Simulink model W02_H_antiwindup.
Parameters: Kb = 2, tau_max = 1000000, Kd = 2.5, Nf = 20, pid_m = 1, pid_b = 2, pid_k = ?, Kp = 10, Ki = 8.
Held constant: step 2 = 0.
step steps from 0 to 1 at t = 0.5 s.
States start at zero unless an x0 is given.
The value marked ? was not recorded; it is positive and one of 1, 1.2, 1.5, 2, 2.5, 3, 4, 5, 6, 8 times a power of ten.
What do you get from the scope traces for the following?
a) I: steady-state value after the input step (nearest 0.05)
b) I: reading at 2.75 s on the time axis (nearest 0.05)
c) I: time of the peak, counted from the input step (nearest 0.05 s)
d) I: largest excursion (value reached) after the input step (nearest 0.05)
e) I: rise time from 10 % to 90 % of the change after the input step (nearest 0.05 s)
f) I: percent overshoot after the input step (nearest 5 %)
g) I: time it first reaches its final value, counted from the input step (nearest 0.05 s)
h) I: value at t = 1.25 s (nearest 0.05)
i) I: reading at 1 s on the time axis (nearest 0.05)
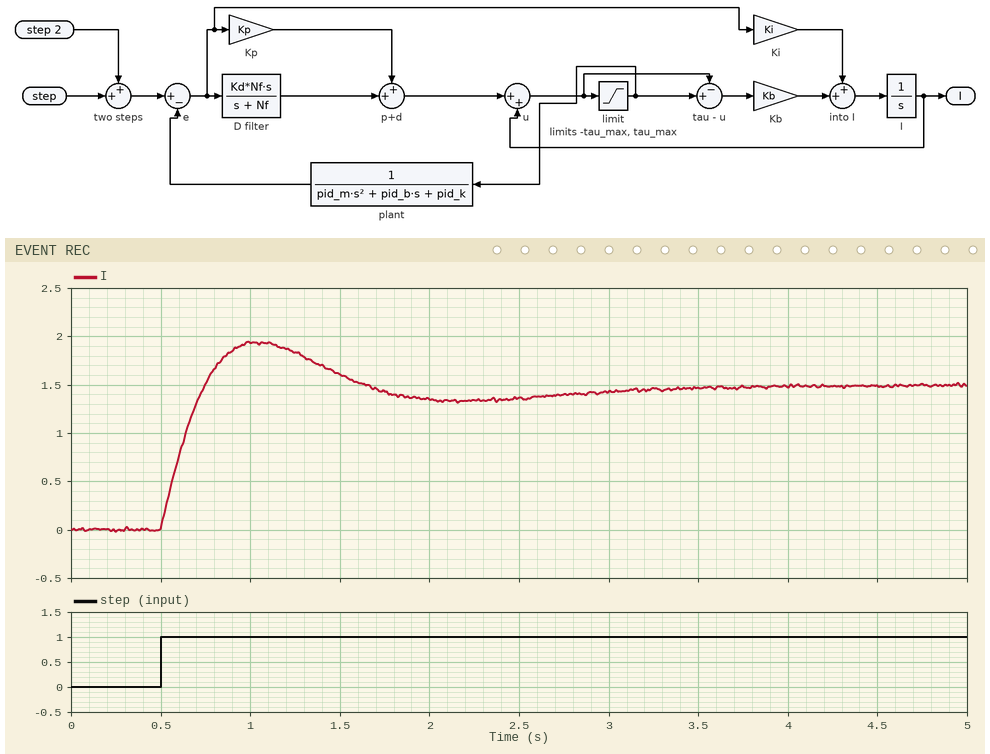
1.50
1.40
0.55 s
1.95
0.20 s
30 %
0.25 s
1.85
1.95
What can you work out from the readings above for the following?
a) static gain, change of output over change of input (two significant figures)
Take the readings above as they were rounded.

1.5
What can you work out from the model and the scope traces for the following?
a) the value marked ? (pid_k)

1.5
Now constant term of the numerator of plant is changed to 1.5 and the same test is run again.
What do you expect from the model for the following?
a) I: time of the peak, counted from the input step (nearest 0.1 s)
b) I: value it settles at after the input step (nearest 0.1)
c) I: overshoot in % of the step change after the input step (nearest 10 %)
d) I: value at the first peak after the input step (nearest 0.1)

0.4 s
1.0
40 %
1.4
